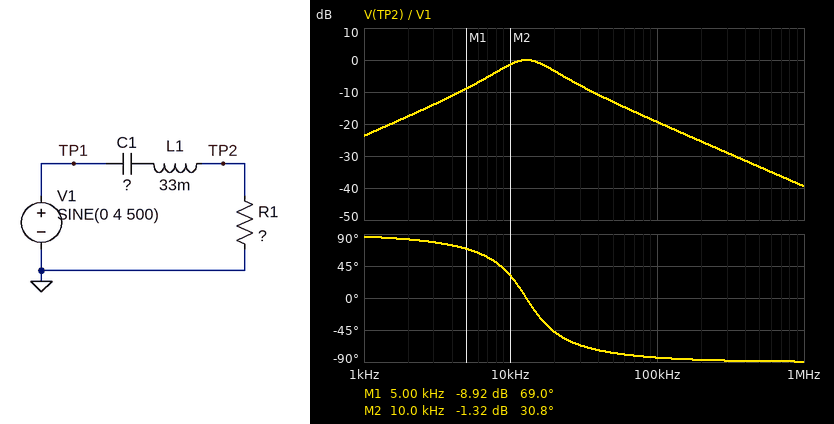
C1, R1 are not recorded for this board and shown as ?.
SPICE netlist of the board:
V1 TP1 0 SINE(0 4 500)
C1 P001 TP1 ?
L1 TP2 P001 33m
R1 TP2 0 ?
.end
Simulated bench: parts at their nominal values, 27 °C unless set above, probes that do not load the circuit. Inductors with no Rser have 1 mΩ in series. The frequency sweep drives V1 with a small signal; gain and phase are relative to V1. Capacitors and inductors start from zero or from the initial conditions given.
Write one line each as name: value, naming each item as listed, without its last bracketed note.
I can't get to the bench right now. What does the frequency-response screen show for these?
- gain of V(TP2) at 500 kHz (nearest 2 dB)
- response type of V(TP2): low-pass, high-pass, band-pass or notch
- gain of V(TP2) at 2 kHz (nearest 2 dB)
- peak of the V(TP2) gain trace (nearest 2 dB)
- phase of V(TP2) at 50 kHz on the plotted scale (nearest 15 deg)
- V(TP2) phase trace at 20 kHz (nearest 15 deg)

gain of V(TP2) at 500 kHz: -34 dB
response type of V(TP2): low-pass, high-pass, band-pass or notch: band-pass
gain of V(TP2) at 2 kHz: -18 dB
peak of the V(TP2) gain trace: 0 dB
phase of V(TP2) at 50 kHz on the plotted scale: -75 deg
V(TP2) phase trace at 20 kHz: -45 deg
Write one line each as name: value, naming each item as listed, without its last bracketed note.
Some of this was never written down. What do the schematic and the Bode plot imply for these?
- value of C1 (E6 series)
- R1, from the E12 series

value of C1: 4.7 nF
R1, from the E12 series: 2.2 kΩ
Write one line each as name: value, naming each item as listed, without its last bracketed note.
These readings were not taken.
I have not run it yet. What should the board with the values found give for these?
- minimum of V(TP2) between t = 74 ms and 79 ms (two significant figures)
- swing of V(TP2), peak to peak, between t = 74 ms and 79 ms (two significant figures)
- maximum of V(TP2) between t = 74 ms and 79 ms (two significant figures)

minimum of V(TP2) between t = 74 ms and 79 ms: -130 mV
swing of V(TP2), peak to peak, between t = 74 ms and 79 ms: 260 mV
maximum of V(TP2) between t = 74 ms and 79 ms: 130 mV
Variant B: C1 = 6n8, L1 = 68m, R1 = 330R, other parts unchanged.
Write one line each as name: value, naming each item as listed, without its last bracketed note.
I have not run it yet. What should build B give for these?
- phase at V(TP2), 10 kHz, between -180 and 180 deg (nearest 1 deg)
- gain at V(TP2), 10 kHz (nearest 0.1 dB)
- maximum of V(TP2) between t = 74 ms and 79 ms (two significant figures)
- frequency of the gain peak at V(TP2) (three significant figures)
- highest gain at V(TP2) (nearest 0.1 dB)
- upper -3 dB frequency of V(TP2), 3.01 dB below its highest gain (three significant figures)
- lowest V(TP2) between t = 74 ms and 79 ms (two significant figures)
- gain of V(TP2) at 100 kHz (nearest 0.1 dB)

phase at V(TP2), 10 kHz, between -180 and 180 deg: -80 deg
gain at V(TP2), 10 kHz: -15.5 dB
maximum of V(TP2) between t = 74 ms and 79 ms: 28 mV
frequency of the gain peak at V(TP2): 7.40 kHz
highest gain at V(TP2): 0 dB
upper -3 dB frequency of V(TP2), 3.01 dB below its highest gain: 7.80 kHz
lowest V(TP2) between t = 74 ms and 79 ms: -28 mV
gain of V(TP2) at 100 kHz: -42.2 dB
